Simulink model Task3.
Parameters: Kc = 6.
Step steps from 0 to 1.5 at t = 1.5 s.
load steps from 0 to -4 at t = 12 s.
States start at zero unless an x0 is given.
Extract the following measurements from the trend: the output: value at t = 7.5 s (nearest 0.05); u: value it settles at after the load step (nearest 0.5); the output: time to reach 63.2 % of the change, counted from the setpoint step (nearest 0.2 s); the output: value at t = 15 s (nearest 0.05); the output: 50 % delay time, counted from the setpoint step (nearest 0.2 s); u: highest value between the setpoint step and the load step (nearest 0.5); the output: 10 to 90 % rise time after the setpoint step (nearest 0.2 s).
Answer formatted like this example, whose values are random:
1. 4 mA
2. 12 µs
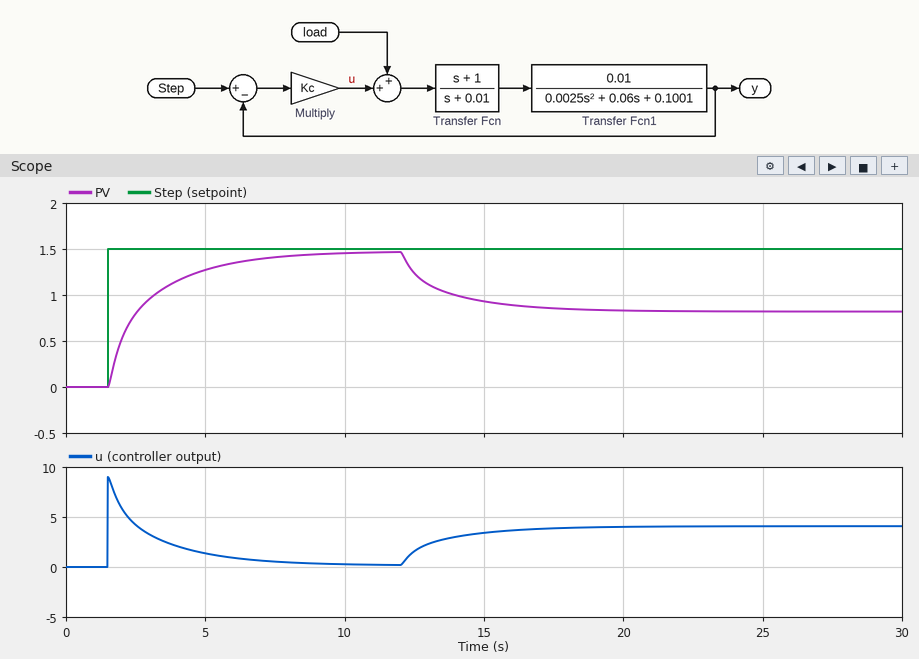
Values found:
1. 1.40
2. 4.0
3. 1.4 s
4. 0.95
5. 0.8 s
6. 9.0
7. 4.0 s
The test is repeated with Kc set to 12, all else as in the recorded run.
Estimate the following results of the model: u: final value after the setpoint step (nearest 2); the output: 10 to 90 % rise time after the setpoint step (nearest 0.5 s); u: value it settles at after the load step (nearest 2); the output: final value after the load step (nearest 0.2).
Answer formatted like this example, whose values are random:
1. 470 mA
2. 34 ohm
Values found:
1. 0
2. 2.0 s
3. 4
4. 1.2
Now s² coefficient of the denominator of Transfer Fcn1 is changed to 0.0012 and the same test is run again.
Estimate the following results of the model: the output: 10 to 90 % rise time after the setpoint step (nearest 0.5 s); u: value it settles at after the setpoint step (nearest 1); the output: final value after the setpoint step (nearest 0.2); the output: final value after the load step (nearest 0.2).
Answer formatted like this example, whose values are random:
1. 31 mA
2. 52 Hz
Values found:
1. 4.0 s
2. 0
3. 1.4
4. 0.8
